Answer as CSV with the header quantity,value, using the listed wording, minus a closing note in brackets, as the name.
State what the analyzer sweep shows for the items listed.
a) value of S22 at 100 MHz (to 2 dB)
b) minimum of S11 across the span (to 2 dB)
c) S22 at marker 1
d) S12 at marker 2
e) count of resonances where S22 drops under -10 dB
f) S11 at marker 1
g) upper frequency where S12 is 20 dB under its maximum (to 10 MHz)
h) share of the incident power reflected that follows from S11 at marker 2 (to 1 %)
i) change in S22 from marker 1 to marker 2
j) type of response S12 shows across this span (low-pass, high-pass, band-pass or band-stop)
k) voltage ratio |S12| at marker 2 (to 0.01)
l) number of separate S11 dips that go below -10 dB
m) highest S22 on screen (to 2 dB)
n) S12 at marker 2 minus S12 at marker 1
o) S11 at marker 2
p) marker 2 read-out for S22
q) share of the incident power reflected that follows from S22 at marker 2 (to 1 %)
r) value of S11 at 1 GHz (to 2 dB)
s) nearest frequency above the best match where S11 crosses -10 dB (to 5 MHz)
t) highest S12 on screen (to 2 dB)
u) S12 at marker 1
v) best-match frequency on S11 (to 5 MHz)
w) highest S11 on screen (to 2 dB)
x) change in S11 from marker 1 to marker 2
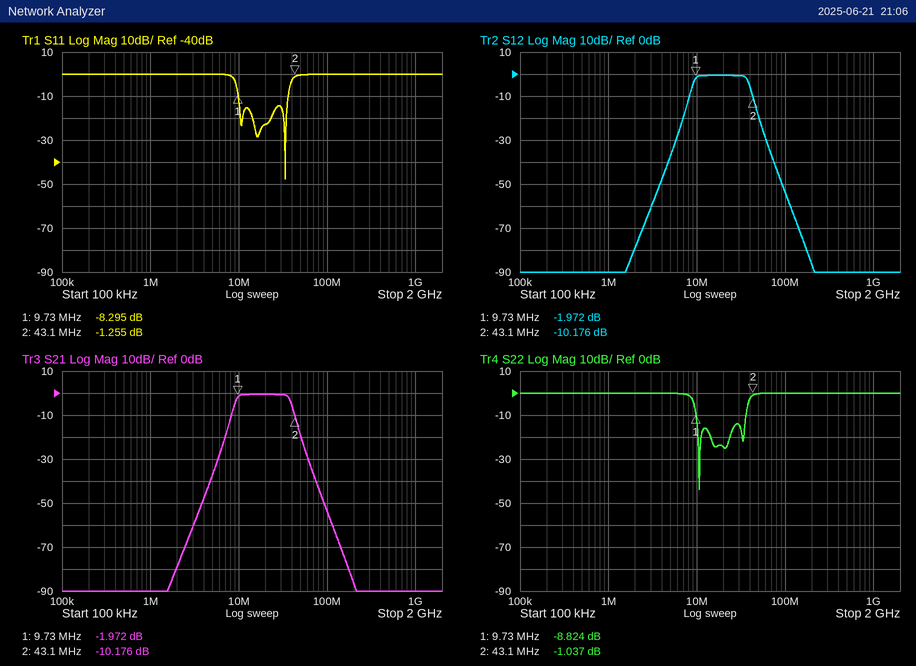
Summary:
quantity,value
value of S22 at 100 MHz,0 dB
minimum of S11 across the span,-48 dB
S22 at marker 1,-8.824 dB
S12 at marker 2,-10.176 dB
count of resonances where S22 drops under -10 dB,3
S11 at marker 1,-8.295 dB
upper frequency where S12 is 20 dB under its maximum,50 MHz
share of the incident power reflected that follows from S11 at marker 2,75 %
change in S22 from marker 1 to marker 2,7.787 dB
type of response S12 shows across this span,band-pass
voltage ratio |S12| at marker 2,0.31
number of separate S11 dips that go below -10 dB,3
highest S22 on screen,0 dB
S12 at marker 2 minus S12 at marker 1,-8.204 dB
S11 at marker 2,-1.255 dB
marker 2 read-out for S22,-1.037 dB
share of the incident power reflected that follows from S22 at marker 2,79 %
value of S11 at 1 GHz,0 dB
nearest frequency above the best match where S11 crosses -10 dB,35 MHz
highest S12 on screen,0 dB
S12 at marker 1,-1.972 dB
best-match frequency on S11,35 MHz
highest S11 on screen,0 dB
change in S11 from marker 1 to marker 2,7.040 dB
